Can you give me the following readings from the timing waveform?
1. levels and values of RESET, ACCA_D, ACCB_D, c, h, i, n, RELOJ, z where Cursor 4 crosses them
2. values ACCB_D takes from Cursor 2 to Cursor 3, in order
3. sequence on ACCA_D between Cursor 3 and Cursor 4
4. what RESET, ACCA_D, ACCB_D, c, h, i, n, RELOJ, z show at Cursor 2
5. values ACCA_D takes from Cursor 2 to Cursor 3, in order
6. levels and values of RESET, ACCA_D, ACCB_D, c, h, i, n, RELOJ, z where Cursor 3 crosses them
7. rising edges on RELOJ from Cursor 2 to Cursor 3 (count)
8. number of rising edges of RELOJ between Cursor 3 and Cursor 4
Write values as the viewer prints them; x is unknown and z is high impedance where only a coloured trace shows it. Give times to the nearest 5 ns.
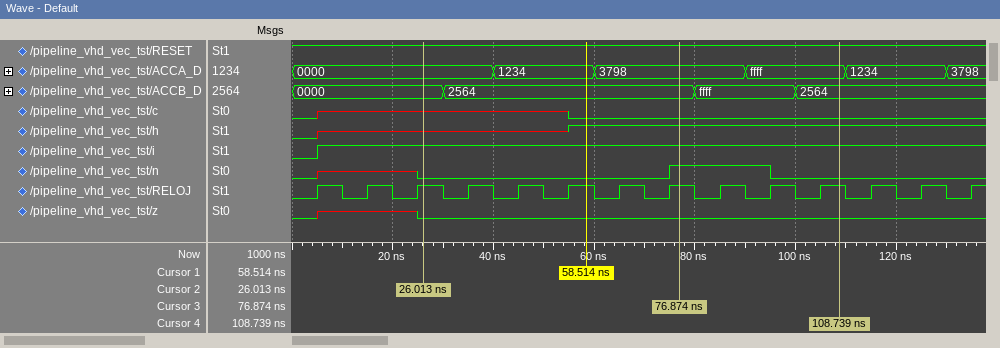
RESET=1, ACCA_D=ffff, ACCB_D=2564, c=0, h=1, i=1, n=0, RELOJ=1, z=0
0000, 2564
3798, ffff
RESET=1, ACCA_D=0000, ACCB_D=0000, c=x, h=x, i=1, n=0, RELOJ=1, z=0
0000, 1234, 3798
RESET=1, ACCA_D=3798, ACCB_D=2564, c=0, h=1, i=1, n=1, RELOJ=1, z=0
5
3
